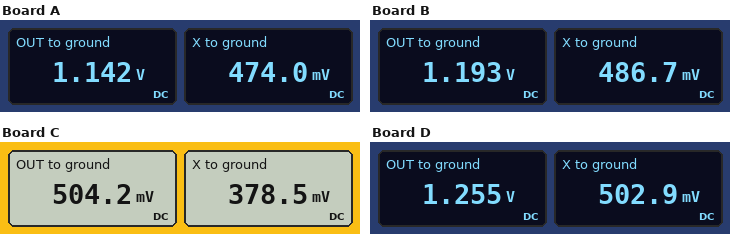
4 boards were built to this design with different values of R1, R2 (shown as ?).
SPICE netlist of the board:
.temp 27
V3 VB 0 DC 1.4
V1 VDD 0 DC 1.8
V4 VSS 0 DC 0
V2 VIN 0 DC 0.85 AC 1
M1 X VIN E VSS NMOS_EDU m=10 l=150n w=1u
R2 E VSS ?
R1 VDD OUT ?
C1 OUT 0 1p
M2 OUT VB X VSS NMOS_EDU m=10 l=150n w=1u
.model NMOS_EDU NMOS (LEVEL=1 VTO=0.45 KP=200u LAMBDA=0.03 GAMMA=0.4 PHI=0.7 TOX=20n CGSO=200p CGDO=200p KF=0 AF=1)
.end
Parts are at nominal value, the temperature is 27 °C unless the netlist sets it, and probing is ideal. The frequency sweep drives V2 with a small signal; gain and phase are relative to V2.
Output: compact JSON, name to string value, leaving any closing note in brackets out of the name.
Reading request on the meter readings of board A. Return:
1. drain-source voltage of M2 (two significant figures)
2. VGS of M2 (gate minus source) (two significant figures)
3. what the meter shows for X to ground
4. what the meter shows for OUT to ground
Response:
{"drain-source voltage of M2": "670 mV", "VGS of M2 (gate minus source)": "930 mV", "what the meter shows for X to ground": "474.0 mV", "what the meter shows for OUT to ground": "1.142 V"}
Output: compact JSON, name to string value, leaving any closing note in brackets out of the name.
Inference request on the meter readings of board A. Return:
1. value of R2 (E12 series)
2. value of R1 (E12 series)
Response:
{"value of R2": "18 Ω", "value of R1": "680 Ω"}
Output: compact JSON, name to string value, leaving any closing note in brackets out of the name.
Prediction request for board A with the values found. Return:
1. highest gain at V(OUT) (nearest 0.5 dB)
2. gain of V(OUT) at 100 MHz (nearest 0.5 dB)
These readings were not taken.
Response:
{"highest gain at V(OUT)": "10.0 dB", "gain of V(OUT) at 100 MHz": "9.0 dB"}
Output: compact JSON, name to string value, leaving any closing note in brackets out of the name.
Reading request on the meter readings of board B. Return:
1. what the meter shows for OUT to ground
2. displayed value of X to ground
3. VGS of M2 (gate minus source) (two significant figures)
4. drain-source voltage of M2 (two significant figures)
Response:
{"what the meter shows for OUT to ground": "1.193 V", "displayed value of X to ground": "486.7 mV", "VGS of M2 (gate minus source)": "910 mV", "drain-source voltage of M2": "710 mV"}
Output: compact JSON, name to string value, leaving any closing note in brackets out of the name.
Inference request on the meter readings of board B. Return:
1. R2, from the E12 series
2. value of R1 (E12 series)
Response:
{"R2, from the E12 series": "33 Ω", "value of R1": "680 Ω"}
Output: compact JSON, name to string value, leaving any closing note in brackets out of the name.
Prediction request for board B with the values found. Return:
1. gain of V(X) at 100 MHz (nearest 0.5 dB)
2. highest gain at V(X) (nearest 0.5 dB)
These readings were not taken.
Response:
{"gain of V(X) at 100 MHz": "-3.0 dB", "highest gain at V(X)": "-3.0 dB"}
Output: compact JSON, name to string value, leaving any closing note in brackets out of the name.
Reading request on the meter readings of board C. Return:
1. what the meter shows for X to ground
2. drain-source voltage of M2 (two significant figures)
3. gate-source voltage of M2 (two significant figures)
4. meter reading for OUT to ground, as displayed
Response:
{"what the meter shows for X to ground": "378.5 mV", "drain-source voltage of M2": "130 mV", "gate-source voltage of M2": "1.0 V", "meter reading for OUT to ground, as displayed": "504.2 mV"}
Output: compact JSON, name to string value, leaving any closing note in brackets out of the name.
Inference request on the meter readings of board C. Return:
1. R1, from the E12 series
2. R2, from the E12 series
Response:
{"R1, from the E12 series": "1.8 kΩ", "R2, from the E12 series": "82 Ω"}
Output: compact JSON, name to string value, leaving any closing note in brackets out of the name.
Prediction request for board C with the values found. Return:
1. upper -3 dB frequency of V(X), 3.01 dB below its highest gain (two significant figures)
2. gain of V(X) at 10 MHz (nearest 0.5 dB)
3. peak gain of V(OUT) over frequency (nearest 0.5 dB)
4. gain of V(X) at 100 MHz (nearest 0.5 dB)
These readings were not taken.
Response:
{"upper -3 dB frequency of V(X), 3.01 dB below its highest gain": "99 MHz", "gain of V(X) at 10 MHz": "11.5 dB", "peak gain of V(OUT) over frequency": "13.5 dB", "gain of V(X) at 100 MHz": "8.5 dB"}
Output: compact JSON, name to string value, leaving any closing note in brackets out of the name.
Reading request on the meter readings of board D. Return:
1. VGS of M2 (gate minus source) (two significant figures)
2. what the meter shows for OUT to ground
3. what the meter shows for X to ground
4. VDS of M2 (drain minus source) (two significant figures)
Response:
{"VGS of M2 (gate minus source)": "900 mV", "what the meter shows for OUT to ground": "1.255 V", "what the meter shows for X to ground": "502.9 mV", "VDS of M2 (drain minus source)": "750 mV"}
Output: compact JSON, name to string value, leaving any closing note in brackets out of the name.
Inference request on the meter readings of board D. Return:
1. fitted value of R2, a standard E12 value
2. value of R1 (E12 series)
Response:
{"fitted value of R2, a standard E12 value": "56 Ω", "value of R1": "680 Ω"}
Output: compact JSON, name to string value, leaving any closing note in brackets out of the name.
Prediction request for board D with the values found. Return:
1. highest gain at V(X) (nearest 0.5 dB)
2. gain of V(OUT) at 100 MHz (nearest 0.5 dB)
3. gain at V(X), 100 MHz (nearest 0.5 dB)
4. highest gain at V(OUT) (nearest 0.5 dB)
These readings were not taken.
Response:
{"highest gain at V(X)": "-4.0 dB", "gain of V(OUT) at 100 MHz": "7.0 dB", "gain at V(X), 100 MHz": "-4.0 dB", "highest gain at V(OUT)": "7.5 dB"}
